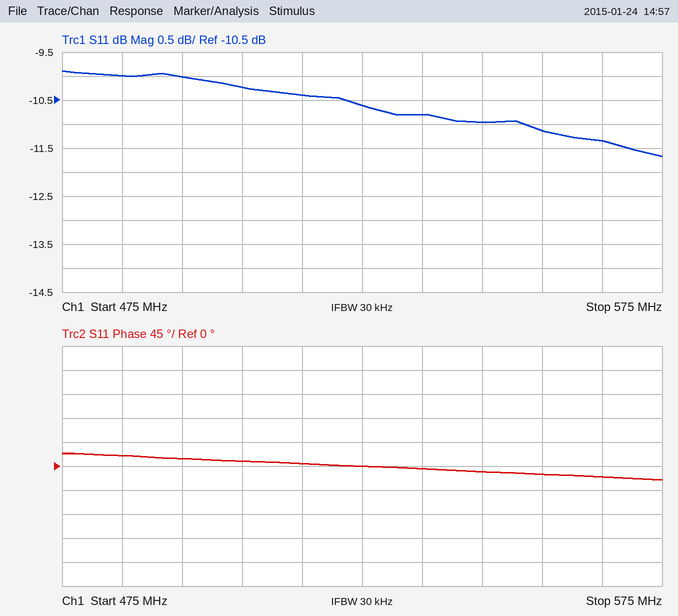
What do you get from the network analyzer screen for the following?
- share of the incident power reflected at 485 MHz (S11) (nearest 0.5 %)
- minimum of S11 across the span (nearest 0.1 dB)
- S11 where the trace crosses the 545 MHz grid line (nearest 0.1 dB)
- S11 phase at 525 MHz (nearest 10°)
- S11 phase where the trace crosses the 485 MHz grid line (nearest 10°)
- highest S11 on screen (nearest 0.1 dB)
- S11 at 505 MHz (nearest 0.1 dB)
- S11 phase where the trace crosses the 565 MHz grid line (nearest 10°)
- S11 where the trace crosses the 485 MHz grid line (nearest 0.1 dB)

10.0 %
-11.7 dB
-11.0 dB
0°
20°
-9.9 dB
-10.2 dB
-20°
-10.0 dB
